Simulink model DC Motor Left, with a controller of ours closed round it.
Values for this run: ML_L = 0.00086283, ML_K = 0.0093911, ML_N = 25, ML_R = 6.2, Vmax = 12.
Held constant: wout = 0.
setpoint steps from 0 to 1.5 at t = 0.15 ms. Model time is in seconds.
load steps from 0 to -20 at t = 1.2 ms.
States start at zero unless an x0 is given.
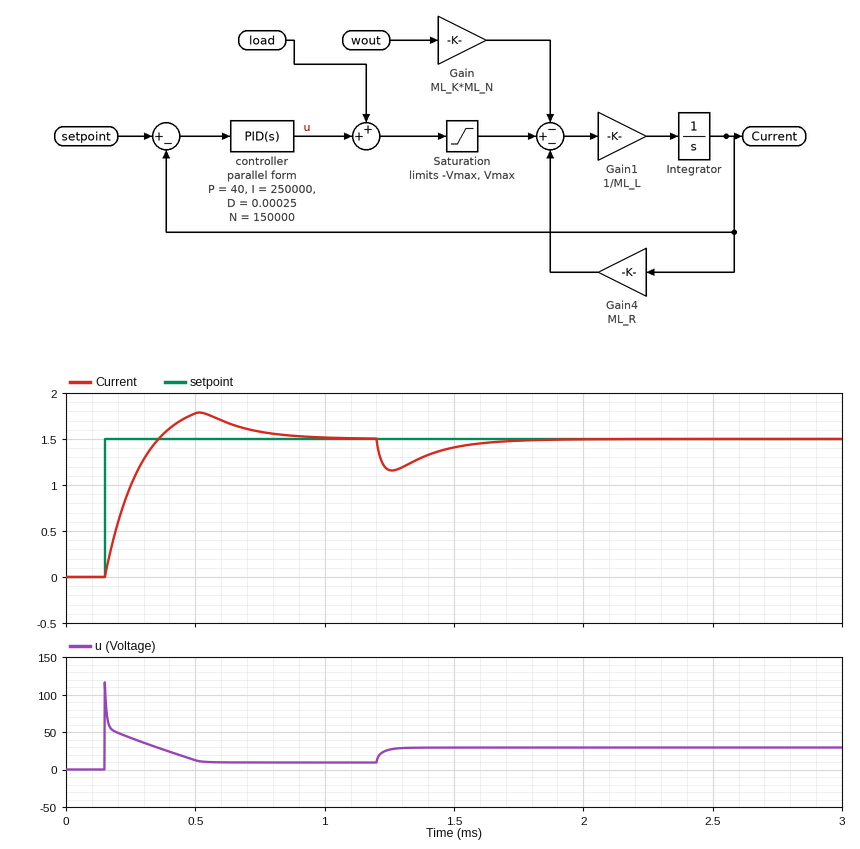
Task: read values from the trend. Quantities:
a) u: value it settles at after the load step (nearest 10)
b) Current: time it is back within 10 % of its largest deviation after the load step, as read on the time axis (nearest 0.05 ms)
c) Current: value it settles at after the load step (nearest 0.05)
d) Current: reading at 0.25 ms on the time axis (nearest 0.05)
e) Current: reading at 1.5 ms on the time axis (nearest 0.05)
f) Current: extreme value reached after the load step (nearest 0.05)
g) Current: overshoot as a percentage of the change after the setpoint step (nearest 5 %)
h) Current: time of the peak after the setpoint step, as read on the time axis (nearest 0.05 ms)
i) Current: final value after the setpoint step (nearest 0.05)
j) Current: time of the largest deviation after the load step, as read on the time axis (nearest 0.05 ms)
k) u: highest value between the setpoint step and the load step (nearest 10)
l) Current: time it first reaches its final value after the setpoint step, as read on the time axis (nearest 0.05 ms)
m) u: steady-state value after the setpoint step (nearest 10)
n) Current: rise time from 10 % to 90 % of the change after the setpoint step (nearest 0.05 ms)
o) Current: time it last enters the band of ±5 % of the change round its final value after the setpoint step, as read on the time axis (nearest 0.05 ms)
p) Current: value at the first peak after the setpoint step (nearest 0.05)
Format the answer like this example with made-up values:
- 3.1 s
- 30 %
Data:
- 30
- 1.65 ms
- 1.50
- 1.00
- 1.40
- 1.15
- 20 %
- 0.50 ms
- 1.50
- 1.25 ms
- 120
- 0.35 ms
- 10
- 0.15 ms
- 0.75 ms
- 1.80
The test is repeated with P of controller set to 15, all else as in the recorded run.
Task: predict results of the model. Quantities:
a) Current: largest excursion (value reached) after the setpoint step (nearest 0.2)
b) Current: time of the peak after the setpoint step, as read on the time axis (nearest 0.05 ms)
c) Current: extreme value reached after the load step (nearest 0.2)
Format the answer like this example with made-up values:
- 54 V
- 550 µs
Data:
- 1.8
- 0.60 ms
- 1.0
